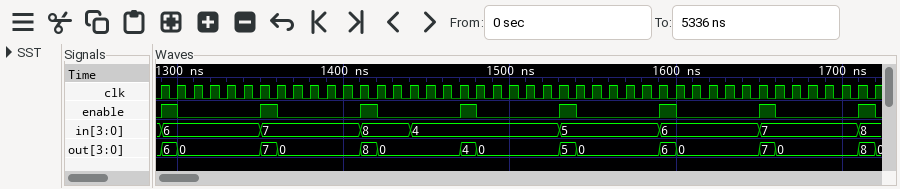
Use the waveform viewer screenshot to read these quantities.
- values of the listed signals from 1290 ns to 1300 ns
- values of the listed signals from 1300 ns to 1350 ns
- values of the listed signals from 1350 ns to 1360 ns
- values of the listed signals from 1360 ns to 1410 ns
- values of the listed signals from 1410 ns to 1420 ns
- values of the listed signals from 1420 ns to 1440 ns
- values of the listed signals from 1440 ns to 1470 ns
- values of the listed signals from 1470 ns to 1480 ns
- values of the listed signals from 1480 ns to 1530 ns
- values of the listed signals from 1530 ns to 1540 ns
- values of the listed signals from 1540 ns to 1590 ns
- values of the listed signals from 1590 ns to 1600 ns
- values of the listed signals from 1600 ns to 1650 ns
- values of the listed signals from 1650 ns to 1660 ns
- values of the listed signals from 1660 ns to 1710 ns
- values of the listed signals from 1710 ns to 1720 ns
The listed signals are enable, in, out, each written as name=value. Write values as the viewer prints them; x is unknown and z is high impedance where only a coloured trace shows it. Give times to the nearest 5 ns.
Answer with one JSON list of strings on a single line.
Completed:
["enable=1, in=6, out=6", "enable=0, in=6, out=0", "enable=1, in=7, out=7", "enable=0, in=7, out=0", "enable=1, in=8, out=8", "enable=0, in=8, out=0", "enable=0, in=4, out=0", "enable=1, in=4, out=4", "enable=0, in=4, out=0", "enable=1, in=5, out=5", "enable=0, in=5, out=0", "enable=1, in=6, out=6", "enable=0, in=6, out=0", "enable=1, in=7, out=7", "enable=0, in=7, out=0", "enable=1, in=8, out=8"]
